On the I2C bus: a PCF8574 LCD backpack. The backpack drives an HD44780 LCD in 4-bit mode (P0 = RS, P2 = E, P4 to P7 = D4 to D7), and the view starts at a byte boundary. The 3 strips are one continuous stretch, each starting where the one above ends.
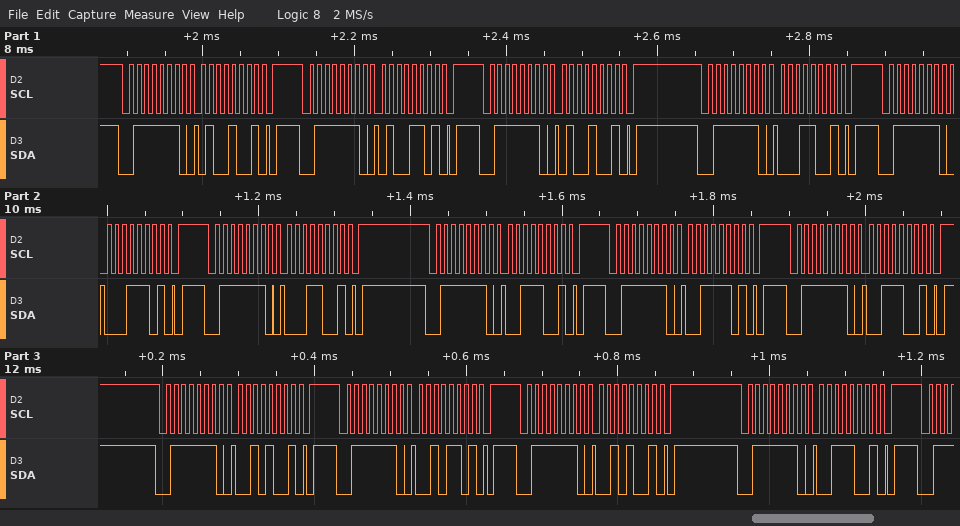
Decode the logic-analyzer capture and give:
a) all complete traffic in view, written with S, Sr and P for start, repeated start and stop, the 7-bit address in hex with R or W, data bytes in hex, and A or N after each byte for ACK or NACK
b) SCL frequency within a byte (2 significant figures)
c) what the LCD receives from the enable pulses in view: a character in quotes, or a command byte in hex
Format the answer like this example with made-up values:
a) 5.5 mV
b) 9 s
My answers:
a) S 3FW A 49 A P S 3FW A 4D A P S 3FW A 49 A P S 3FW A 19 A P S 3FW A 1D A P S 3FW A 19 A P S 3FW A 39 A P S 3FW A 3D A P S 3FW A 39 A P S 3FW A 29 A P S 3FW A 2D A P S 3FW A 29 A P S 3FW A 39 A P
b) 100 kHz
c) 'A' '2'
